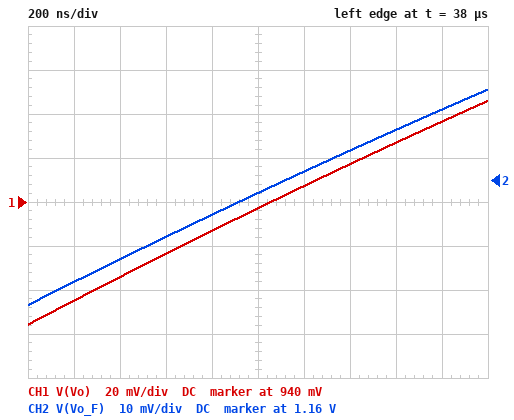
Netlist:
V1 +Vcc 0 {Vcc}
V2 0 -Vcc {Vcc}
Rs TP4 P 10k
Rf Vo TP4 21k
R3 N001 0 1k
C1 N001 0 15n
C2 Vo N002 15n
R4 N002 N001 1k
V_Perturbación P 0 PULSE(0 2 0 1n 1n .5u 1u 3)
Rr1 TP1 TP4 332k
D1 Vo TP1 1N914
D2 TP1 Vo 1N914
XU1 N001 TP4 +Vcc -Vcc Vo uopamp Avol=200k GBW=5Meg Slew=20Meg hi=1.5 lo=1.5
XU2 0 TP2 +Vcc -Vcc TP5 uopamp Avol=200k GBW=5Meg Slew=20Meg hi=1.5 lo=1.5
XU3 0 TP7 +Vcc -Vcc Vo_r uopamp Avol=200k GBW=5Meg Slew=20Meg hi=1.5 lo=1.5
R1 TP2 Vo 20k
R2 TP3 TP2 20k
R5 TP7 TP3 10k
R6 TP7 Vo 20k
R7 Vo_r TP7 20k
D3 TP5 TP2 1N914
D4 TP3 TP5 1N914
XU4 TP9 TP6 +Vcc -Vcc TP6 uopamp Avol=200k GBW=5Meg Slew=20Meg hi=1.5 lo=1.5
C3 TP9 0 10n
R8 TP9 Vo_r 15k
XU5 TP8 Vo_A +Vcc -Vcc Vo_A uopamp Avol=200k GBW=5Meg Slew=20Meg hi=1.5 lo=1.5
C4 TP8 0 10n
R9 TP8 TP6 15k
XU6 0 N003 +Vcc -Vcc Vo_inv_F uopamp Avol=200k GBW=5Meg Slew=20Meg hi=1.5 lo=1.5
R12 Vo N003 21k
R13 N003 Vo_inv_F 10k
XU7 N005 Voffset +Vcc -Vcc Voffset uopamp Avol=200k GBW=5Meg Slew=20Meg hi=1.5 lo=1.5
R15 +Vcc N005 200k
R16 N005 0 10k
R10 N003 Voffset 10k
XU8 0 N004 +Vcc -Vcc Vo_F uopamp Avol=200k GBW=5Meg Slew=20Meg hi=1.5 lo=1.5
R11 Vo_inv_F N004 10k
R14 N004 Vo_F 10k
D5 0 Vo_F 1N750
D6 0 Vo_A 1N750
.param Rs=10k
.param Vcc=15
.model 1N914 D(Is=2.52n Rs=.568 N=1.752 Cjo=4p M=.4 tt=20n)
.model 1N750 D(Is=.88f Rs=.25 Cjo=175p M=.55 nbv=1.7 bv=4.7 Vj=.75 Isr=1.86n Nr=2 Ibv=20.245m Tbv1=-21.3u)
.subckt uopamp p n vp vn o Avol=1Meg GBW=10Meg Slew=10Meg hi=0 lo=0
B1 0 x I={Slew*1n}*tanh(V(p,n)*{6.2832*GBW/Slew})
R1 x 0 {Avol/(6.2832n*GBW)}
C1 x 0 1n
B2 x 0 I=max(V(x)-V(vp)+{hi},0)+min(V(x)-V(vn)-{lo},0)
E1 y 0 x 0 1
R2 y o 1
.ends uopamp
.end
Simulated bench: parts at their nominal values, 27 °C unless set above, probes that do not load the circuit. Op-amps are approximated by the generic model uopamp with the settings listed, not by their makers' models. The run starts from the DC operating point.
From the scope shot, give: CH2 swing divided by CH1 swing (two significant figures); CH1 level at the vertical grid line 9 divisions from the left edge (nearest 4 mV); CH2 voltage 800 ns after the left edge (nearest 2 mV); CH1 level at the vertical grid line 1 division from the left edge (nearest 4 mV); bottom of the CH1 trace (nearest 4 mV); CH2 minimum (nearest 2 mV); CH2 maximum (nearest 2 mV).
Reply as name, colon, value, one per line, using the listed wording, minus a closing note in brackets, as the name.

CH2 swing divided by CH1 swing: 0.48
CH1 level at the vertical grid line 9 divisions from the left edge: 976 mV
CH2 voltage 800 ns after the left edge: 1.152 V
CH1 level at the vertical grid line 1 division from the left edge: 896 mV
bottom of the CH1 trace: 884 mV
CH2 minimum: 1.132 V
CH2 maximum: 1.180 V
